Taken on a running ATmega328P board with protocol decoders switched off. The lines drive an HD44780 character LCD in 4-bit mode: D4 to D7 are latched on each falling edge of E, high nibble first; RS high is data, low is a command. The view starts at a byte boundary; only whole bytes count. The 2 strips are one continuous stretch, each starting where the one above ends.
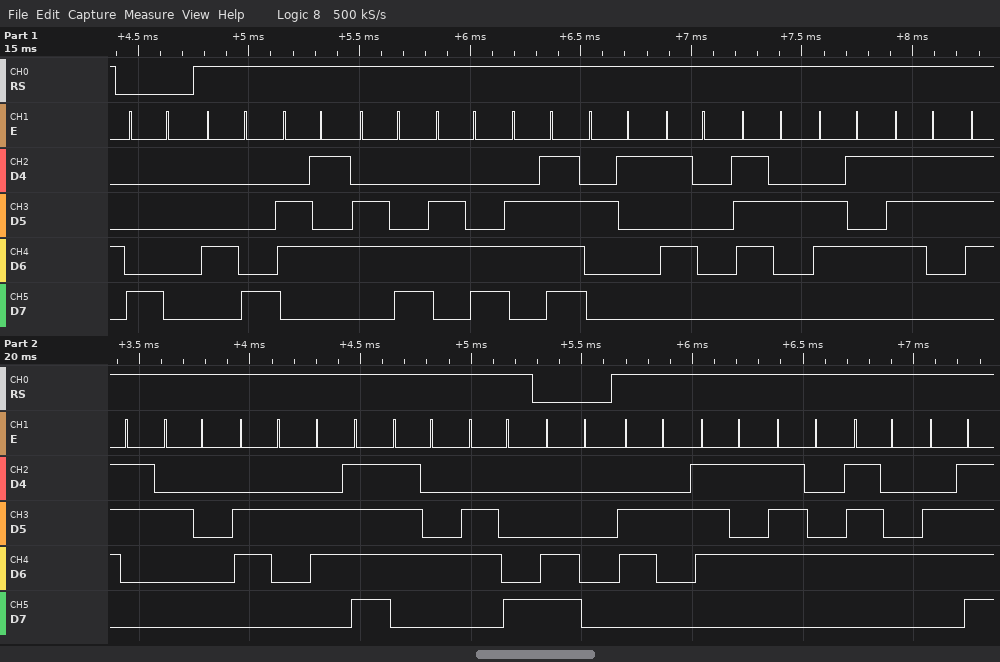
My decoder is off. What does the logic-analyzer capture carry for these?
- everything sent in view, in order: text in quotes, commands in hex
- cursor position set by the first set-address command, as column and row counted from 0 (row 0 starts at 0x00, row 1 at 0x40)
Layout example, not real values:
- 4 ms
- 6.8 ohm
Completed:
- 0x80 "Hello!Press both" 0xC0 "butto"
- column 0, row 0
